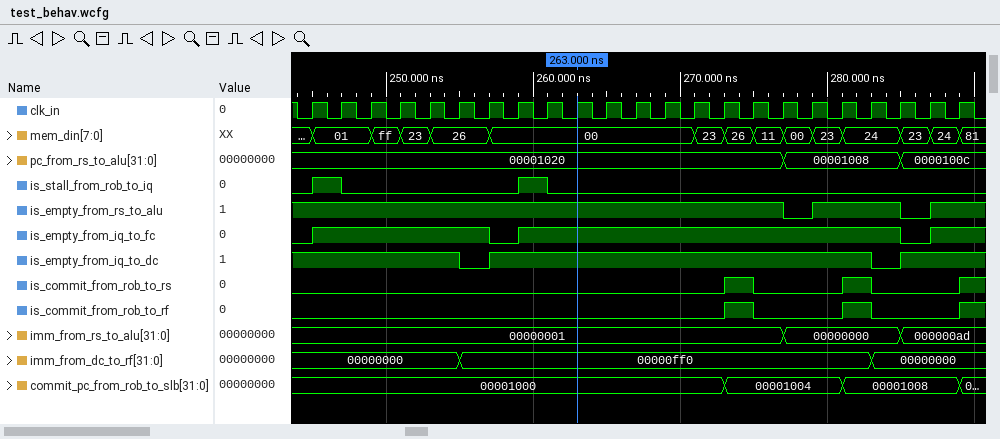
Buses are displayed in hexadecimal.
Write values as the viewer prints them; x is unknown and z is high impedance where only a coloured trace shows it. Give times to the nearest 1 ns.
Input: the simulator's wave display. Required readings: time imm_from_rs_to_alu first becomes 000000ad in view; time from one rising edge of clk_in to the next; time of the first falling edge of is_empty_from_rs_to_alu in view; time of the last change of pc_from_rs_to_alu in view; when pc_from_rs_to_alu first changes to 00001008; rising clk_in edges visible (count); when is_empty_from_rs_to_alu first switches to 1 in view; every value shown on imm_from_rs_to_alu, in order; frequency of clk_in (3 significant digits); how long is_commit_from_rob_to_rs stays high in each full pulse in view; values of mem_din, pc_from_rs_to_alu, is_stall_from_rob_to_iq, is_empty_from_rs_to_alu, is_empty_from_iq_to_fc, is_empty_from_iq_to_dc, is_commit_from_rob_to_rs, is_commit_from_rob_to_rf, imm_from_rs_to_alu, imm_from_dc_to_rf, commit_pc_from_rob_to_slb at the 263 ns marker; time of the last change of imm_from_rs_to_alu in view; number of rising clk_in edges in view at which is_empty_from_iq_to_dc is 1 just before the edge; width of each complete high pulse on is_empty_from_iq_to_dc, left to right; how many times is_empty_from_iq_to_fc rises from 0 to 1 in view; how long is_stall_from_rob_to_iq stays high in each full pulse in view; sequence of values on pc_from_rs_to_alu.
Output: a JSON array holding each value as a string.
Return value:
["285 ns", "2 ns", "277 ns", "285 ns", "277 ns", "23", "279 ns", "00000001, 00000000, 000000ad", "500 MHz", "2 ns, 2 ns", "mem_din=00, pc_from_rs_to_alu=00001020, is_stall_from_rob_to_iq=0, is_empty_from_rs_to_alu=1, is_empty_from_iq_to_fc=1, is_empty_from_iq_to_dc=1, is_commit_from_rob_to_rs=0, is_commit_from_rob_to_rf=0, imm_from_rs_to_alu=00000001, imm_from_dc_to_rf=00000ff0, commit_pc_from_rob_to_slb=00001000", "285 ns", "21", "26 ns", "3", "2 ns, 2 ns", "00001020, 00001008, 0000100c"]
